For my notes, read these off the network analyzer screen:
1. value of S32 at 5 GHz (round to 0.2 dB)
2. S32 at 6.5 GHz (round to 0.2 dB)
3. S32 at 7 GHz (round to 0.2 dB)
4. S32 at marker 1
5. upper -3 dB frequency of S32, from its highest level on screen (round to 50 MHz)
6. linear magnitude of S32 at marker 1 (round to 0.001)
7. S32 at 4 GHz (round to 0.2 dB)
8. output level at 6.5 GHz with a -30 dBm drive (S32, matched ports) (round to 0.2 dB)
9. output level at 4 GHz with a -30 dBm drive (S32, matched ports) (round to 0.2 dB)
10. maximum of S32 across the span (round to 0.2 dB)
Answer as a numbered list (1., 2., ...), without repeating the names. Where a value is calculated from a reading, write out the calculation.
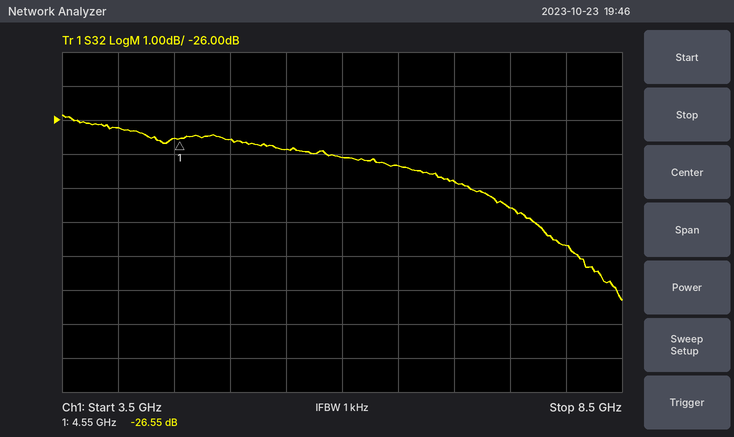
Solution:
1. -26.6 dB
2. -27.4 dB
3. -27.8 dB
4. -26.55 dB
5. 7.65 GHz
6. 10^(-26.55/20) ≈ 0.047
7. -26.2 dB
8. -30 dBm + (-27.4 dB) = -57.4 dBm
9. -30 dBm + (-26.2 dB) = -56.2 dBm
10. -25.8 dB
